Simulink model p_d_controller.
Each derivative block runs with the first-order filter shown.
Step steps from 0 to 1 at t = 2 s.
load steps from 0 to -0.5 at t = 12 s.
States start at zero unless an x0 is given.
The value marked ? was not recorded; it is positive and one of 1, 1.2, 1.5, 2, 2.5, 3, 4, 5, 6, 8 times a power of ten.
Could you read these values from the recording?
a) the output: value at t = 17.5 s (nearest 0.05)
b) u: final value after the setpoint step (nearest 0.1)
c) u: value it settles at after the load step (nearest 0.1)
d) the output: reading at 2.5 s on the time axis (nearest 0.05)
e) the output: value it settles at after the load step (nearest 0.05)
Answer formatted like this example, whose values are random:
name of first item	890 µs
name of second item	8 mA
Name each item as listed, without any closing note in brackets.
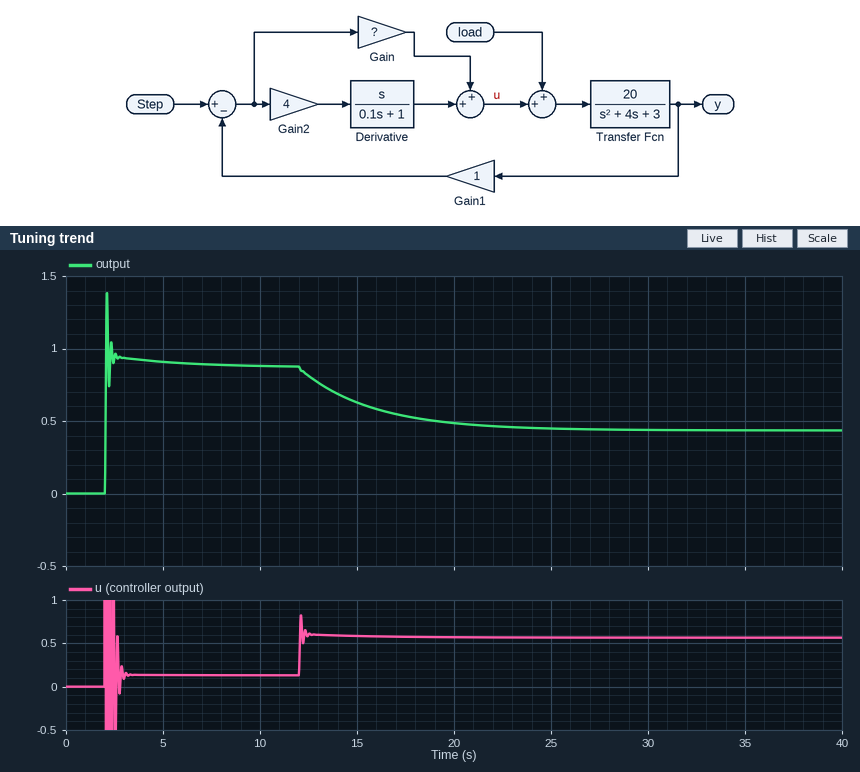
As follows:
the output: value at t = 17.5 s	0.55
u: final value after the setpoint step	0.1
u: value it settles at after the load step	0.6
the output: reading at 2.5 s on the time axis	0.95
the output: value it settles at after the load step	0.45
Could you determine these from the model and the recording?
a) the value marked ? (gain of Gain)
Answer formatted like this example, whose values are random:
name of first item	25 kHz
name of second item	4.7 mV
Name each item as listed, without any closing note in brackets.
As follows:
the value marked ?	1
